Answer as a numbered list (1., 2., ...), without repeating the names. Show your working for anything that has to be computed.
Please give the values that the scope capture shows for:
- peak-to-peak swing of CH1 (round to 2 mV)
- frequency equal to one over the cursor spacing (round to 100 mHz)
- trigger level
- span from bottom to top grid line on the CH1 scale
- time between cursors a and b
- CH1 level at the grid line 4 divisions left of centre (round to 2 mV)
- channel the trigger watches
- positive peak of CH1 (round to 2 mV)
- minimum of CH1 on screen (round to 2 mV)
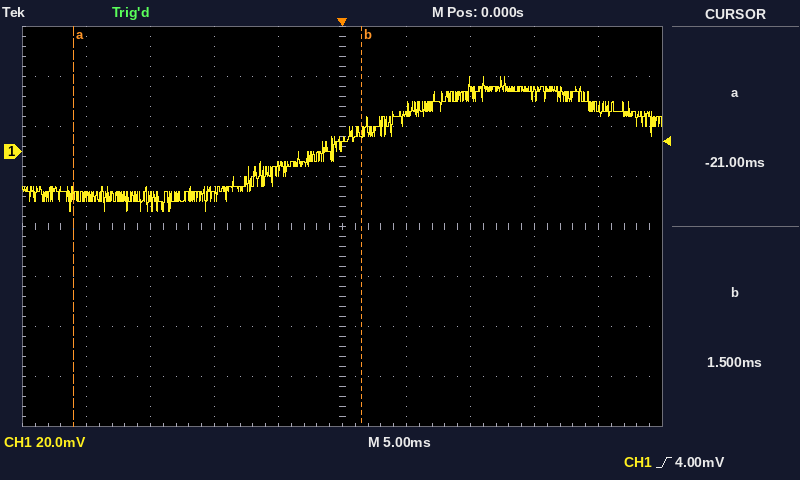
1. 30 mV − (-24 mV) = 54 mV
2. 1 / 22.5 ms ≈ 44.4 Hz
3. 4.00 mV
4. 160 mV
5. 1.5 ms − (-21 ms) = 22.5 ms
6. -18 mV
7. CH1
8. 30 mV
9. -24 mV
